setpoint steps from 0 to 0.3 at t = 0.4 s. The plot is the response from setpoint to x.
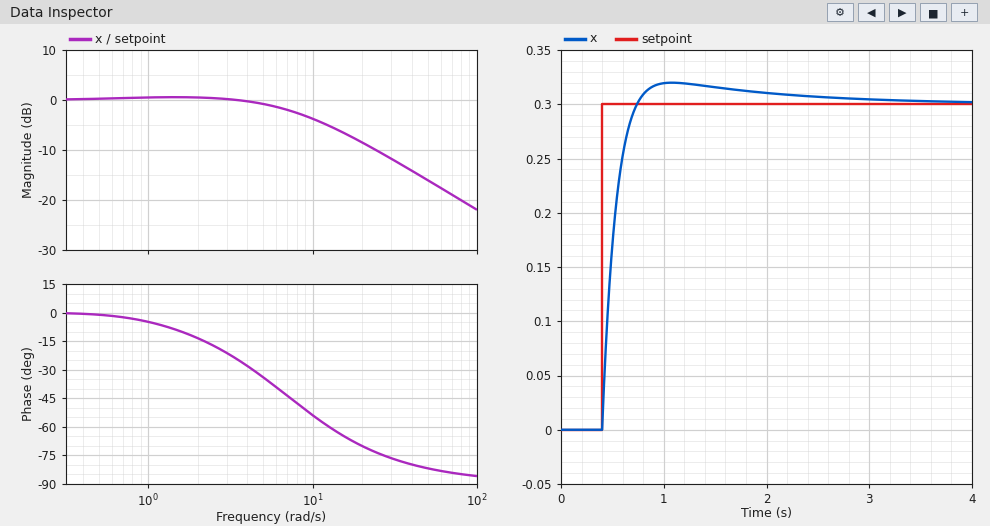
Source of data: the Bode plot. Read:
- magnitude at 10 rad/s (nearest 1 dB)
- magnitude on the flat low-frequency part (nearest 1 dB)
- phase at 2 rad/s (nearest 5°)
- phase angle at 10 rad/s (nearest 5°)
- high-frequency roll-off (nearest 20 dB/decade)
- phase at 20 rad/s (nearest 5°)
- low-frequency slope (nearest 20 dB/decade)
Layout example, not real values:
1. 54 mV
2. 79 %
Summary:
1. -4 dB
2. 0 dB
3. -15°
4. -55°
5. -20 dB/decade
6. -70°
7. 0 dB/decade
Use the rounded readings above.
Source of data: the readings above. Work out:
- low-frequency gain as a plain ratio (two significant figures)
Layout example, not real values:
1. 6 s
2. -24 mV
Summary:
1. 1.0
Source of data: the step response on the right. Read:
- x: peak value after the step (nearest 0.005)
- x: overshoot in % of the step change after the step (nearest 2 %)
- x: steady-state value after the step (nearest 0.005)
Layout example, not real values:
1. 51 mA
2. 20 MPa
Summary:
1. 0.320
2. 6 %
3. 0.300
